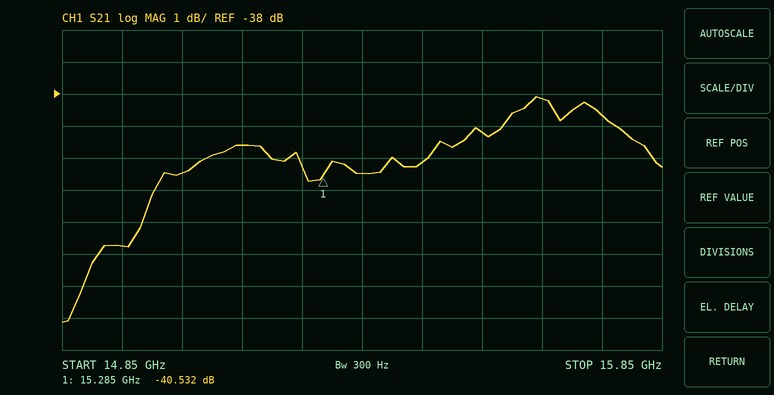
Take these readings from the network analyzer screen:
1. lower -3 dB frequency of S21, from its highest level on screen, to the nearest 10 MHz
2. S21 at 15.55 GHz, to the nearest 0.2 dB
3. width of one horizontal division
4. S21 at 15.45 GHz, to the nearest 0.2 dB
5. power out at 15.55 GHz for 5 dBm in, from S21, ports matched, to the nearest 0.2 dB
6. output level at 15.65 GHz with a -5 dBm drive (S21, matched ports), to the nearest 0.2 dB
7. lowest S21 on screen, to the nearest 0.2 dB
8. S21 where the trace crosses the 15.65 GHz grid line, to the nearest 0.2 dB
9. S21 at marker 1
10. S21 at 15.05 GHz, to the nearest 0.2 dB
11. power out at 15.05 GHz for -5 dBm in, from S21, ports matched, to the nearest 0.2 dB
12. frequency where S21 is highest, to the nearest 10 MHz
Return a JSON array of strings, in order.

["15.00 GHz", "-39.2 dB", "100 MHz", "-40.2 dB", "-34.2 dBm", "-43.2 dBm", "-45.2 dB", "-38.2 dB", "-40.532 dB", "-40.4 dB", "-45.4 dBm", "15.64 GHz"]
